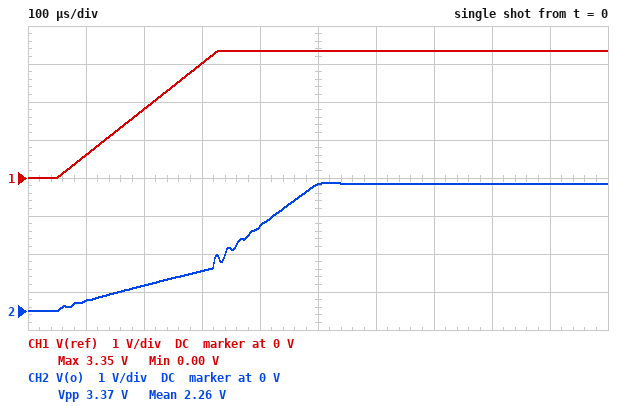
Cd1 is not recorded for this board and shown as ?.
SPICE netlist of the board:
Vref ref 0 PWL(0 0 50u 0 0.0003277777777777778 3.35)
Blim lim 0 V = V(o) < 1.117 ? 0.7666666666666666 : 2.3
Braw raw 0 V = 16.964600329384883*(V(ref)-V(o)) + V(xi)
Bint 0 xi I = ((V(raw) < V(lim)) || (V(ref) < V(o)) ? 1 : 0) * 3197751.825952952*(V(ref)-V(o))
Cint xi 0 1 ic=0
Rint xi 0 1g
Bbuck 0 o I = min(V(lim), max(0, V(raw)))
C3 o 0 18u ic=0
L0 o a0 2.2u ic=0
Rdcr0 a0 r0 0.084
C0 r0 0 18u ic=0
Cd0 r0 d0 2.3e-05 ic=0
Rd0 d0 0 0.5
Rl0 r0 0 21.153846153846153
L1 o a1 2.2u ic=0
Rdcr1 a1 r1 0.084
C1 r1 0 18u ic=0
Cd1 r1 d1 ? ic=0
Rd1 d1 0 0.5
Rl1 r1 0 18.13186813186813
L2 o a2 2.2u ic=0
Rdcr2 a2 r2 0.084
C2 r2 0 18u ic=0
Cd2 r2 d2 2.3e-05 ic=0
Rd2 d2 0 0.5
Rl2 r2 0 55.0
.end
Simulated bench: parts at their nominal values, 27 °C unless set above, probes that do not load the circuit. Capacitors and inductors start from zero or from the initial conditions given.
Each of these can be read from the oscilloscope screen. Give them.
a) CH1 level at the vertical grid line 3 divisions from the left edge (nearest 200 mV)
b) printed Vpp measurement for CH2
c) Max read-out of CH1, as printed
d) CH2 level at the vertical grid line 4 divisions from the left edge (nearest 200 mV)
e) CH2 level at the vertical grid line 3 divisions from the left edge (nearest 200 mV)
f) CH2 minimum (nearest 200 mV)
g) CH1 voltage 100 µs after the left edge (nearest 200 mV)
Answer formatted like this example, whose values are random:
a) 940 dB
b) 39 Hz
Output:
a) 3.0 V
b) 3.37 V
c) 3.35 V
d) 2.2 V
e) 1.0 V
f) 0 V
g) 600 mV
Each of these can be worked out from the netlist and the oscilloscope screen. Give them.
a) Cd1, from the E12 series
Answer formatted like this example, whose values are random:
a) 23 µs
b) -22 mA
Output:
a) 56 µF
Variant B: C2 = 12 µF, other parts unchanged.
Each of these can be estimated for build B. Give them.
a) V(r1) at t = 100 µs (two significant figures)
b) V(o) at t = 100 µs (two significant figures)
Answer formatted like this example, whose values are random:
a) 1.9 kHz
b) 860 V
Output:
a) 240 mV
b) 280 mV
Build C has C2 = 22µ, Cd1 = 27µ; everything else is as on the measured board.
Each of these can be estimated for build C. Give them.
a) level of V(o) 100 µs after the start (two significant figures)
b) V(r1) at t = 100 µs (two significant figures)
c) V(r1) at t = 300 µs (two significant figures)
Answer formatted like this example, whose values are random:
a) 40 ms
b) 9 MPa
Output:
a) 280 mV
b) 250 mV
c) 1.4 V
